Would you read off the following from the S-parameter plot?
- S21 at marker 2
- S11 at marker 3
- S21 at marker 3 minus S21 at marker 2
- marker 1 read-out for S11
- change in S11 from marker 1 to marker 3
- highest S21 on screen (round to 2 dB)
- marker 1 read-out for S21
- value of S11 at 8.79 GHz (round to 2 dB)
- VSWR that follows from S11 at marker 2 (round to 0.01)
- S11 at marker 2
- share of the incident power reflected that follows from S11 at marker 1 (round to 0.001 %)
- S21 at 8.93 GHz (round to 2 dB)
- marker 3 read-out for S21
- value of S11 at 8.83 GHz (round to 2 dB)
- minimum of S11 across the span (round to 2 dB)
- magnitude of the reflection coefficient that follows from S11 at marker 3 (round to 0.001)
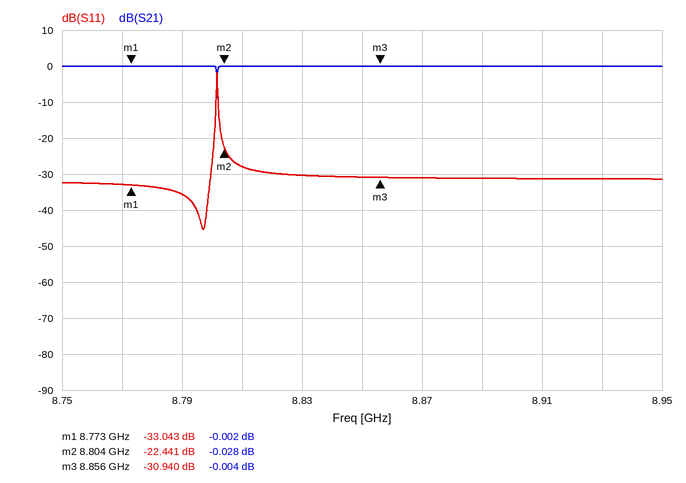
-0.028 dB
-30.940 dB
0.024 dB
-33.043 dB
2.103 dB
0 dB
-0.002 dB
-36 dB
1.16
-22.441 dB
0.050 %
0 dB
-0.004 dB
-30 dB
-46 dB
0.028
